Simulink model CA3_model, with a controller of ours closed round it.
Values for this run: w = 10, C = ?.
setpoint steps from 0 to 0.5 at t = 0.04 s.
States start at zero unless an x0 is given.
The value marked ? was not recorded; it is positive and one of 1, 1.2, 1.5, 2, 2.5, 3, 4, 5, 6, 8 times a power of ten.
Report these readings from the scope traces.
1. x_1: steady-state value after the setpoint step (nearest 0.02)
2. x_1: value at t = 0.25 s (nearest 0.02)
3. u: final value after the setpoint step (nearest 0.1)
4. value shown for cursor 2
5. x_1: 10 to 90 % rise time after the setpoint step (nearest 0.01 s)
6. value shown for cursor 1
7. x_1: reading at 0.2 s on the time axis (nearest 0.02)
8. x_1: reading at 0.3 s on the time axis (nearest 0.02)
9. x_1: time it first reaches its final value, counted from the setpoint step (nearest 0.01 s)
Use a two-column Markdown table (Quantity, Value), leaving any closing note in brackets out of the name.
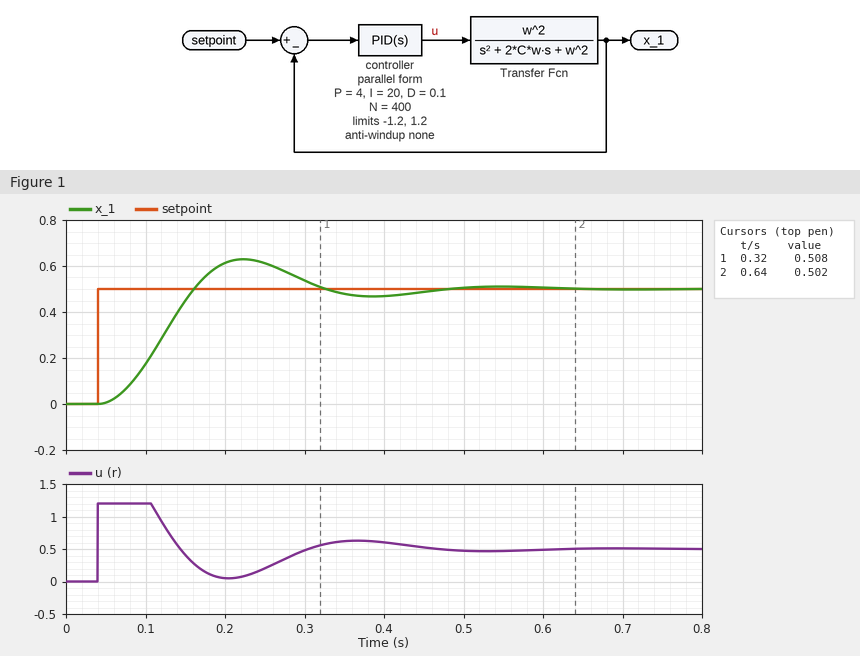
| Quantity | Value |
|---|---|
| x_1: steady-state value after the setpoint step | 0.50 |
| x_1: value at t = 0.25 s | 0.62 |
| u: final value after the setpoint step | 0.5 |
| value shown for cursor 2 | 0.502 |
| x_1: 10 to 90 % rise time after the setpoint step | 0.08 s |
| value shown for cursor 1 | 0.508 |
| x_1: reading at 0.2 s on the time axis | 0.62 |
| x_1: reading at 0.3 s on the time axis | 0.54 |
| x_1: time it first reaches its final value, counted from the setpoint step | 0.12 s |
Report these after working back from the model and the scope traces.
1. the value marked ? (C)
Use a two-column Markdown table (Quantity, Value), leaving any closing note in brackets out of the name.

| Quantity | Value |
|---|---|
| the value marked ? | 0.5 |
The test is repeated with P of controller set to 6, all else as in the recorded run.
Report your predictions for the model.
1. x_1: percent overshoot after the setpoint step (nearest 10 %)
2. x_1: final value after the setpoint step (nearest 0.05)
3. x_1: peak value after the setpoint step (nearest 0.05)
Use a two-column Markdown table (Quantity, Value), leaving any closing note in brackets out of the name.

| Quantity | Value |
|---|---|
| x_1: percent overshoot after the setpoint step | 30 % |
| x_1: final value after the setpoint step | 0.50 |
| x_1: peak value after the setpoint step | 0.65 |
